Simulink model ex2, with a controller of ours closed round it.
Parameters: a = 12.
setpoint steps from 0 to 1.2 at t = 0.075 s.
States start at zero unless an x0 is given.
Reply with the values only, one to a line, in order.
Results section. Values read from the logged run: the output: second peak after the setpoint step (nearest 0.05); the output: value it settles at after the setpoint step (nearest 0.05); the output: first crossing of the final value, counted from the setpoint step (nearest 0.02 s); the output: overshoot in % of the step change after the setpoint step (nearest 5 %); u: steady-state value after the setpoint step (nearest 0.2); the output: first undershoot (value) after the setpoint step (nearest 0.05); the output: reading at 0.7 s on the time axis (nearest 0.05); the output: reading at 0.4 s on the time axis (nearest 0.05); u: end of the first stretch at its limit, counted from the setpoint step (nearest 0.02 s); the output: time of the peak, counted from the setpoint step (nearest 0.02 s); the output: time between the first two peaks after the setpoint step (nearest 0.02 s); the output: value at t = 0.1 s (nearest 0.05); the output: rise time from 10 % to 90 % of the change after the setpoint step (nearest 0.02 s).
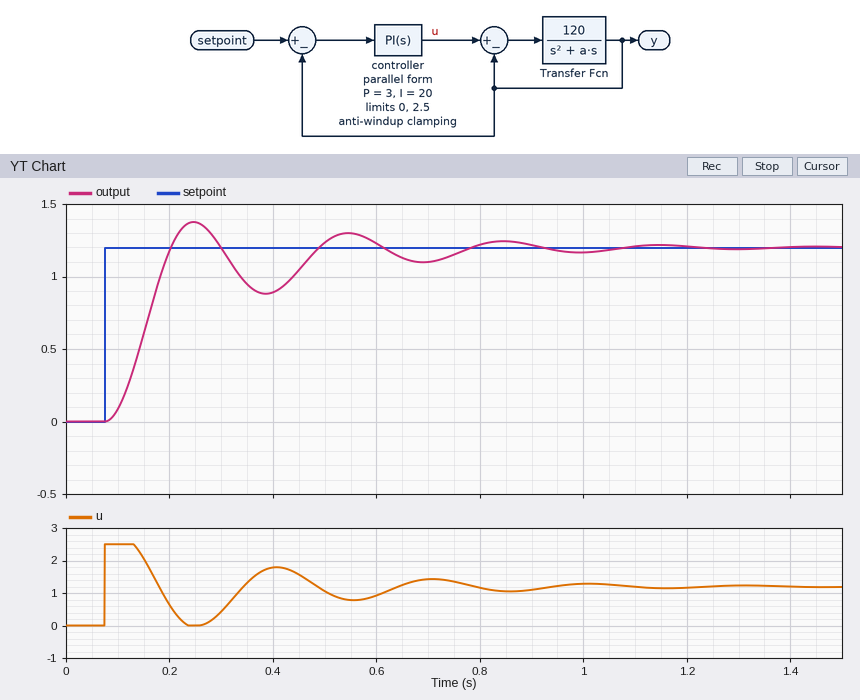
1.30
1.20
0.12 s
15 %
1.2
0.90
1.10
0.90
0.06 s
0.18 s
0.30 s
0.10
0.08 s
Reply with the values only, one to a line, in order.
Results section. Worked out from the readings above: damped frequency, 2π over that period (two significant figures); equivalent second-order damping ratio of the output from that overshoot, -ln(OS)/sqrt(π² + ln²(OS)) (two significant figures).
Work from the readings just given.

21 rad/s
0.52
